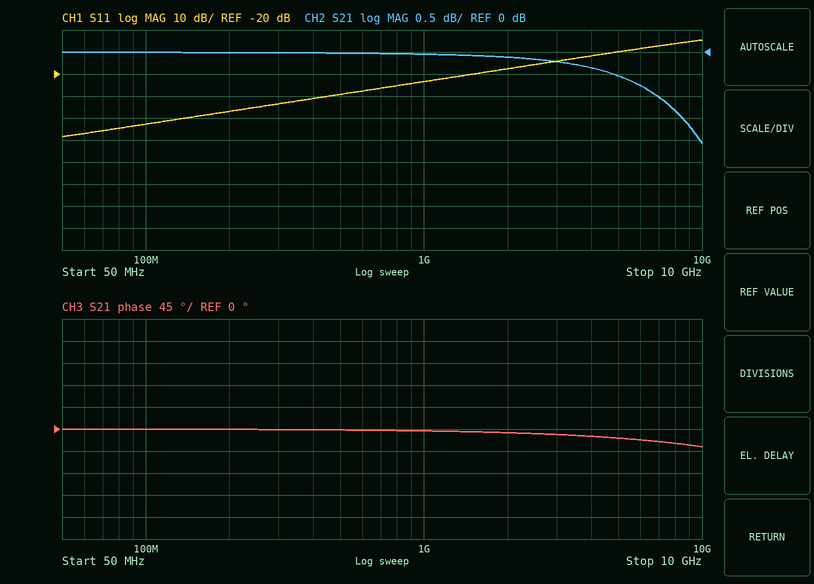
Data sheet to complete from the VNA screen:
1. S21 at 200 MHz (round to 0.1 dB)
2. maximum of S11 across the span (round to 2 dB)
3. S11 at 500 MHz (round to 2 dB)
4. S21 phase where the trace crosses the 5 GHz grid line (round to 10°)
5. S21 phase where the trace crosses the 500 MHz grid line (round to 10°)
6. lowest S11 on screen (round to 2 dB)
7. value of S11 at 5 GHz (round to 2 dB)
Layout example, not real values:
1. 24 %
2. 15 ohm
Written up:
1. 0.0 dB
2. -4 dB
3. -30 dB
4. -20°
5. 0°
6. -48 dB
7. -10 dB
